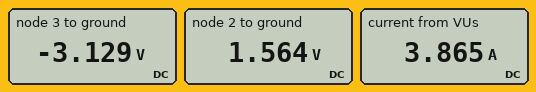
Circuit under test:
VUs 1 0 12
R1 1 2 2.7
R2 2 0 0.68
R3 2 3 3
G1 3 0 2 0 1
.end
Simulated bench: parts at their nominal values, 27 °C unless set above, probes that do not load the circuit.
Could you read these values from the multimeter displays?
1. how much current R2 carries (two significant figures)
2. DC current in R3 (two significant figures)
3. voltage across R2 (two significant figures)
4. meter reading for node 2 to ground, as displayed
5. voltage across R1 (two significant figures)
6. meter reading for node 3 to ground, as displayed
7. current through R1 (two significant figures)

2.3 A
1.6 A
1.6 V
1.564 V
10 V
-3.129 V
3.9 A
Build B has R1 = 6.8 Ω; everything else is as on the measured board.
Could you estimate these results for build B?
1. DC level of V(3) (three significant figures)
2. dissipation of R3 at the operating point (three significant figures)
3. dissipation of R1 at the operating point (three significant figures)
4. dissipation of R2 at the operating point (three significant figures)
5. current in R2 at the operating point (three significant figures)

-1.35 V
1.36 W
18.9 W
668 mW
991 mA
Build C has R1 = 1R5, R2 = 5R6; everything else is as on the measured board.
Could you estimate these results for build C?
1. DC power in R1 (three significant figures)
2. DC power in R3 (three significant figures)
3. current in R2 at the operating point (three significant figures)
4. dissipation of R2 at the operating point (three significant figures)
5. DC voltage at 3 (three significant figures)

39.2 W
56.4 W
774 mA
3.36 W
-8.67 V
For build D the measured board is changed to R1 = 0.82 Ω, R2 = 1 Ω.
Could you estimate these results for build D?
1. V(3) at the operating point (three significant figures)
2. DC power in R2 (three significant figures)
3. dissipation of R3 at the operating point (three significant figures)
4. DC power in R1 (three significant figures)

-9.09 V
20.7 W
62.0 W
67.8 W
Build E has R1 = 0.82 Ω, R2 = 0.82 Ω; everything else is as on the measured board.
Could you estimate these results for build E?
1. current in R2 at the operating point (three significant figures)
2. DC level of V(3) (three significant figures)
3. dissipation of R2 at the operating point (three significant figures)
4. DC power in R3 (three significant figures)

5.19 A
-8.51 V
22.1 W
54.3 W
